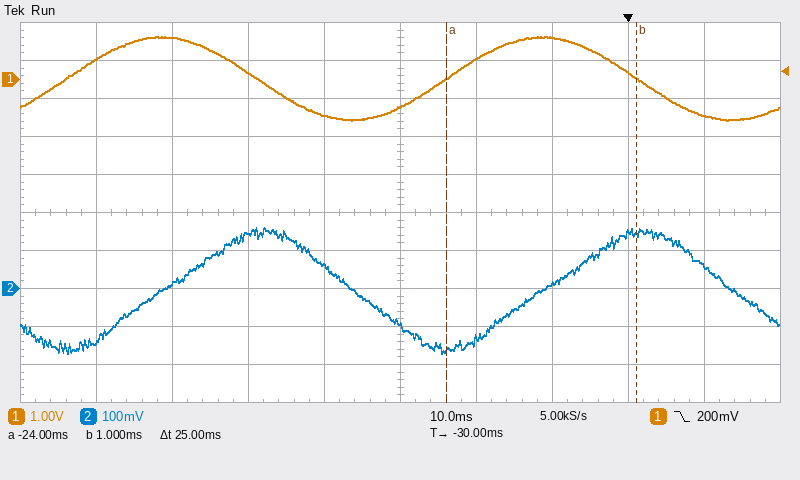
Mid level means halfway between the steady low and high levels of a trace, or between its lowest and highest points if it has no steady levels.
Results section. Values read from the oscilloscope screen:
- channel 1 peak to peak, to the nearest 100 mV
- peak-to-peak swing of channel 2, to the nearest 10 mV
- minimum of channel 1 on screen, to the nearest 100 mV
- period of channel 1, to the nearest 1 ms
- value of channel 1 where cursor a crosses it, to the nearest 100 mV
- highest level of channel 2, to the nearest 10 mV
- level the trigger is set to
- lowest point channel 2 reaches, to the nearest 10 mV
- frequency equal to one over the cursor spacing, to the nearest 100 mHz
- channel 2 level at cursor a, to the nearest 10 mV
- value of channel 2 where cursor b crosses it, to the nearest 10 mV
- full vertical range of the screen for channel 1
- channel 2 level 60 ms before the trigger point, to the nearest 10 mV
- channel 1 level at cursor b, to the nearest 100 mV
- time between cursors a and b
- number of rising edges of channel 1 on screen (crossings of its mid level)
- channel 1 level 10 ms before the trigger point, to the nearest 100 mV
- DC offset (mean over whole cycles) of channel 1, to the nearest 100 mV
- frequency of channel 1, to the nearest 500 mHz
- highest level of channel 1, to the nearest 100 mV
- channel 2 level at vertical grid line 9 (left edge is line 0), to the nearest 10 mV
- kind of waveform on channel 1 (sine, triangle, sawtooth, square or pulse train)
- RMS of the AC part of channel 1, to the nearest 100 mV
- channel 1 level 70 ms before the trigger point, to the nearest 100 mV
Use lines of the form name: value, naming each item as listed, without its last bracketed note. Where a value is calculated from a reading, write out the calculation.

channel 1 peak to peak, to the nearest 100 mV: 1.1 V − (-1.1 V) = 2.2 V
peak-to-peak swing of channel 2, to the nearest 10 mV: 160 mV − (-170 mV) = 330 mV
minimum of channel 1 on screen, to the nearest 100 mV: -1.1 V
period of channel 1, to the nearest 1 ms: 50 ms
value of channel 1 where cursor a crosses it, to the nearest 100 mV: 0.0 V
highest level of channel 2, to the nearest 10 mV: 160 mV
level the trigger is set to: 200 mV
lowest point channel 2 reaches, to the nearest 10 mV: -170 mV
frequency equal to one over the cursor spacing, to the nearest 100 mHz: 1 / 25 ms ≈ 40.0 Hz
channel 2 level at cursor a, to the nearest 10 mV: -160 mV
value of channel 2 where cursor b crosses it, to the nearest 10 mV: 150 mV
full vertical range of the screen for channel 1: 10 V
channel 2 level 60 ms before the trigger point, to the nearest 10 mV: 10 mV
channel 1 level at cursor b, to the nearest 100 mV: 0.0 V
time between cursors a and b: 25 ms
number of rising edges of channel 1 on screen: 2
channel 1 level 10 ms before the trigger point, to the nearest 100 mV: 1.1 V
DC offset (mean over whole cycles) of channel 1, to the nearest 100 mV: (1.1 V + (-1.1 V)) / 2 ≈ 0.0 V
frequency of channel 1, to the nearest 500 mHz: 1 / 50 ms ≈ 20.0 Hz
highest level of channel 1, to the nearest 100 mV: 1.1 V
channel 2 level at vertical grid line 9 (left edge is line 0), to the nearest 10 mV: 60 mV
kind of waveform on channel 1: sine
RMS of the AC part of channel 1, to the nearest 100 mV: 2.2 V / (2√2) ≈ 778 mV, so 800 mV to the nearest 100 mV
channel 1 level 70 ms before the trigger point, to the nearest 100 mV: 500 mV
